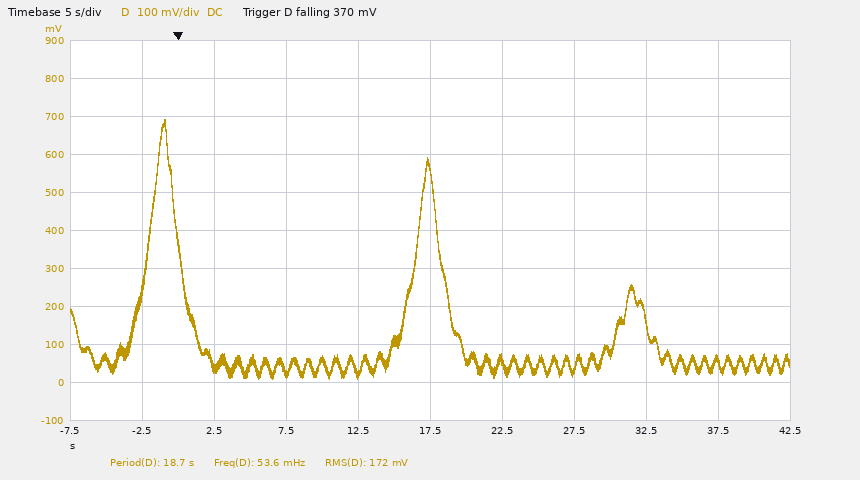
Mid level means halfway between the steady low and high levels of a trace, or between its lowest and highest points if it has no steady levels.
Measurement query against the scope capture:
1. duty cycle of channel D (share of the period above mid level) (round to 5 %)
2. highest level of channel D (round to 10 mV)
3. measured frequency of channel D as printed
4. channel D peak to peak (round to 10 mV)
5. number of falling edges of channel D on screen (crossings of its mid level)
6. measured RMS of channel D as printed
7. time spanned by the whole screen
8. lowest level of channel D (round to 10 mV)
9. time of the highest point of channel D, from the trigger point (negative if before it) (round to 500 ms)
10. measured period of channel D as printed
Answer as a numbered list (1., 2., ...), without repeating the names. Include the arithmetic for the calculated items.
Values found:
1. 10 %
2. 690 mV
3. 53.6 mHz
4. 690 mV − (10 mV) = 680 mV
5. 2
6. 172 mV
7. 50 s
8. 10 mV
9. -1.0 s
10. 18.7 s
